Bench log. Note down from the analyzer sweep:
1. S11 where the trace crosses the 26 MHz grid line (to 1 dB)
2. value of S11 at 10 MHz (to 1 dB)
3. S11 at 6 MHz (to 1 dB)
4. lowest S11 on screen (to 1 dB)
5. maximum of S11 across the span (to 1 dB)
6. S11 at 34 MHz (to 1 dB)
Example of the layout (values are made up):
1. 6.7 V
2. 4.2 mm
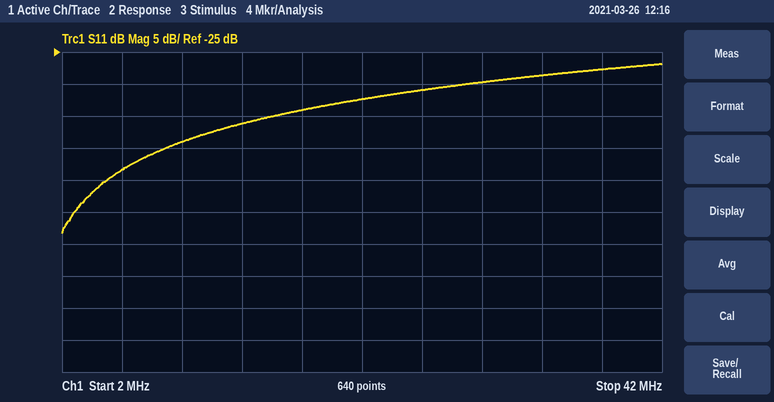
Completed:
1. -31 dB
2. -39 dB
3. -43 dB
4. -53 dB
5. -27 dB
6. -29 dB
